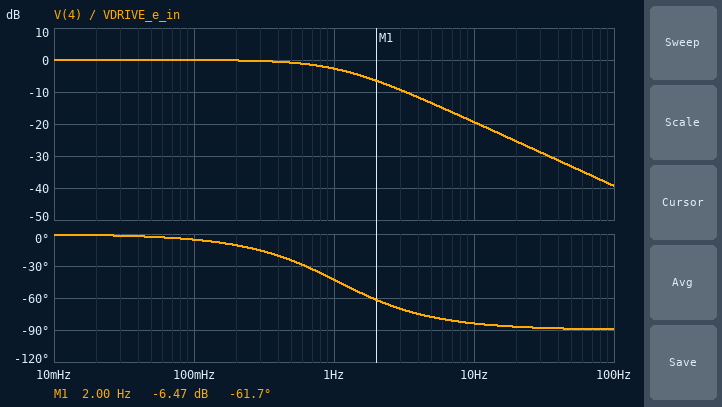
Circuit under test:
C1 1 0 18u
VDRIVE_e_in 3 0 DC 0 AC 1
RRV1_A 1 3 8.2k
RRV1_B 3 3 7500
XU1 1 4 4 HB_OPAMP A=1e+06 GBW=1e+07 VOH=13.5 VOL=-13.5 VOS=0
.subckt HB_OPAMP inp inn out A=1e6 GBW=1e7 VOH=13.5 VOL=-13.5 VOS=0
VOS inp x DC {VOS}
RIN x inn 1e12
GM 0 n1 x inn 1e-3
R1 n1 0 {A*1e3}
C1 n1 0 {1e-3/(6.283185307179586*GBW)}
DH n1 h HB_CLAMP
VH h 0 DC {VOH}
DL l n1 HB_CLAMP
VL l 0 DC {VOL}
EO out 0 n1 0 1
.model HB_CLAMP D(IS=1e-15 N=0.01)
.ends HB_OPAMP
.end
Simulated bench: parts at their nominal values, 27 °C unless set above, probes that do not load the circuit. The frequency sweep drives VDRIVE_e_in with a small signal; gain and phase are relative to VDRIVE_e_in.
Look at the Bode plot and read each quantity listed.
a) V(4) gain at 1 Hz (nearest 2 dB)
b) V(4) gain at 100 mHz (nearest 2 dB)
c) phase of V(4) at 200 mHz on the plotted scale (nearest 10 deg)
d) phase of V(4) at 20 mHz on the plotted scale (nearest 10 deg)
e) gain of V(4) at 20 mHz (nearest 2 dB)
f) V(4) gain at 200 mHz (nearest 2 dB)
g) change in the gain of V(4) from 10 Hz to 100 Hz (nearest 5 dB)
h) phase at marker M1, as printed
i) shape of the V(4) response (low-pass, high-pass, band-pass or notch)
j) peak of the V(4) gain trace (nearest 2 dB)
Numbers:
-2 dB
0 dB
-10 deg
0 deg
0 dB
0 dB
-20 dB
-61.7 deg
low-pass
0 dB
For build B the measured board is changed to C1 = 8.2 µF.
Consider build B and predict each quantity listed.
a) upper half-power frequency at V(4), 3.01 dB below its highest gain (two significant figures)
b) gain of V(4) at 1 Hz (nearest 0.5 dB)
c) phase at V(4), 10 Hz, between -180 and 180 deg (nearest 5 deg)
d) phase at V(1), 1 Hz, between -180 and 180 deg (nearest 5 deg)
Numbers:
2.4 Hz
-0.5 dB
-75 deg
-25 deg
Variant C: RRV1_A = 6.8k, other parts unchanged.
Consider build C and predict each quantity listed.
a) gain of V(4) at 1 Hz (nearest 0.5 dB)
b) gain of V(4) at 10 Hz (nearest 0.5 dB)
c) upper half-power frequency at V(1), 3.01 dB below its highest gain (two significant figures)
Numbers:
-2.0 dB
-18.0 dB
1.3 Hz
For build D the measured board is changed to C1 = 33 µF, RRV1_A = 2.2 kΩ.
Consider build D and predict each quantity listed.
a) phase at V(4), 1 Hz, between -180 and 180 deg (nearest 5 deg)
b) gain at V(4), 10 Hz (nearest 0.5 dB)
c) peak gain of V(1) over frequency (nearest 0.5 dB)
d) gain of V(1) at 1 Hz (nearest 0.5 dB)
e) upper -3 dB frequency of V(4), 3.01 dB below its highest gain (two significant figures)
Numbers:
-25 deg
-13.5 dB
0 dB
-1.0 dB
2.2 Hz
